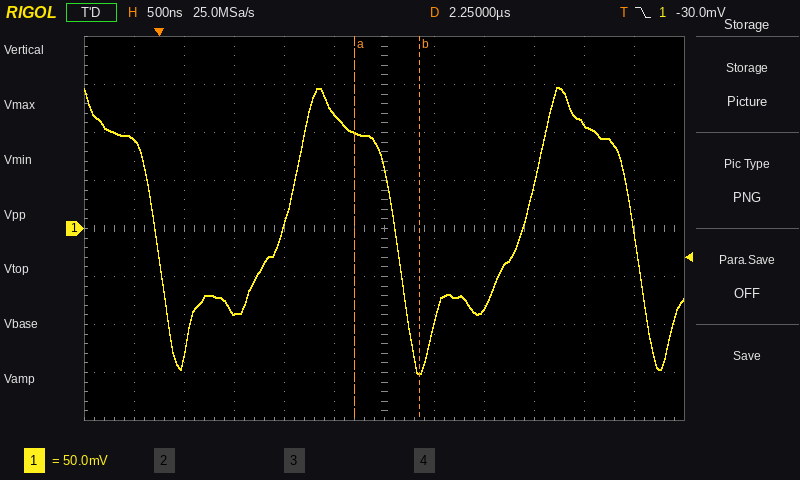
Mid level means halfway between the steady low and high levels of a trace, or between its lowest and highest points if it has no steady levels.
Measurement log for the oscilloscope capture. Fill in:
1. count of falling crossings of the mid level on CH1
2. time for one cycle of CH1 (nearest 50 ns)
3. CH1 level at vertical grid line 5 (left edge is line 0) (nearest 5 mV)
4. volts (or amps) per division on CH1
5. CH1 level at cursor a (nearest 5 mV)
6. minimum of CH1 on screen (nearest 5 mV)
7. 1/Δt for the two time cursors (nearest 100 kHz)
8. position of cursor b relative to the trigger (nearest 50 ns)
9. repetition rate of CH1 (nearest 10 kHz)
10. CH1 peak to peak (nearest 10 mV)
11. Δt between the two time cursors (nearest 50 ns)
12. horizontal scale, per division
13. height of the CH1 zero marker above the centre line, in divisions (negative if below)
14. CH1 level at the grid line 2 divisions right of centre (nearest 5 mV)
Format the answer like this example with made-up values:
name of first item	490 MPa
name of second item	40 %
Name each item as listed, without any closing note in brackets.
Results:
count of falling crossings of the mid level on CH1	3
time for one cycle of CH1	2.40 µs
CH1 level at vertical grid line 5 (left edge is line 0)	120 mV
volts (or amps) per division on CH1	50 mV
CH1 level at cursor a	100 mV
minimum of CH1 on screen	-150 mV
1/Δt for the two time cursors	1.5 MHz
position of cursor b relative to the trigger	+2.60 µs
repetition rate of CH1	420 kHz
CH1 peak to peak	300 mV
Δt between the two time cursors	650 ns
horizontal scale, per division	500 ns
height of the CH1 zero marker above the centre line, in divisions	0.0 div
CH1 level at the grid line 2 divisions right of centre	-85 mV
